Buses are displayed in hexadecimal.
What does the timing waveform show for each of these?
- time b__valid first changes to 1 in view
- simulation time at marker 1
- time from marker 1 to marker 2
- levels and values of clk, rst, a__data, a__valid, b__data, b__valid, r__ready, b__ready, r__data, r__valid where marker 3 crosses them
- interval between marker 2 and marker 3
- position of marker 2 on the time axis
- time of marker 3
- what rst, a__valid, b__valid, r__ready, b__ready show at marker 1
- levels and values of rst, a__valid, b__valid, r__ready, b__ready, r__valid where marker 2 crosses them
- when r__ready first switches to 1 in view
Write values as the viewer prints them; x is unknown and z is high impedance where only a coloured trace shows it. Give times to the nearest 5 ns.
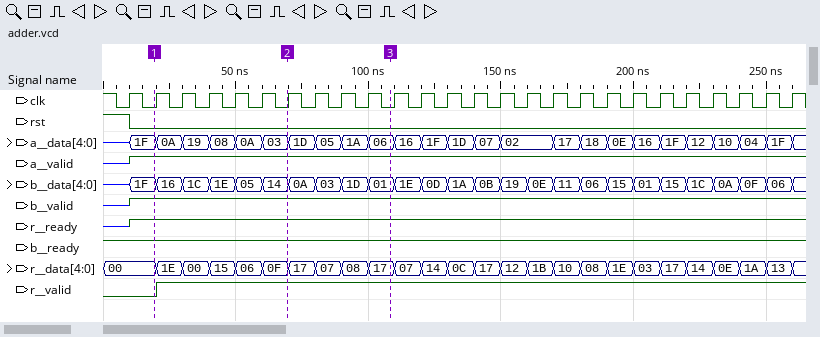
10 ns
20 ns
50 ns
clk=0, rst=0, a__data=06, a__valid=1, b__data=01, b__valid=1, r__ready=1, b__ready=1, r__data=17, r__valid=1
40 ns
70 ns
110 ns
rst=0, a__valid=1, b__valid=1, r__ready=1, b__ready=1
rst=0, a__valid=1, b__valid=1, r__ready=1, b__ready=1, r__valid=1
10 ns
